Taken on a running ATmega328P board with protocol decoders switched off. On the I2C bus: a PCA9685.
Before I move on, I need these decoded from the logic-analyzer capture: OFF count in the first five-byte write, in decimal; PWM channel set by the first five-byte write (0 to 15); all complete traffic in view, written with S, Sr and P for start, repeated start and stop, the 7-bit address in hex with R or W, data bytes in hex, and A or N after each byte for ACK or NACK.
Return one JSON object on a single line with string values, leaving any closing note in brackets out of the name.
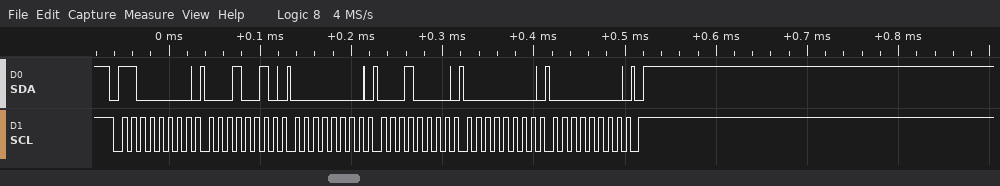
{"OFF count in the first five-byte write, in decimal": "0", "PWM channel set by the first five-byte write": "3", "all complete traffic in view, written with S, Sr and P for start, repeated start and stop, the 7-bit address in hex with R or W, data bytes in hex, and A or N after each byte for ACK or NACK": "S 60W A 12 A 00 A 10 A 00 A 00 A P"}
